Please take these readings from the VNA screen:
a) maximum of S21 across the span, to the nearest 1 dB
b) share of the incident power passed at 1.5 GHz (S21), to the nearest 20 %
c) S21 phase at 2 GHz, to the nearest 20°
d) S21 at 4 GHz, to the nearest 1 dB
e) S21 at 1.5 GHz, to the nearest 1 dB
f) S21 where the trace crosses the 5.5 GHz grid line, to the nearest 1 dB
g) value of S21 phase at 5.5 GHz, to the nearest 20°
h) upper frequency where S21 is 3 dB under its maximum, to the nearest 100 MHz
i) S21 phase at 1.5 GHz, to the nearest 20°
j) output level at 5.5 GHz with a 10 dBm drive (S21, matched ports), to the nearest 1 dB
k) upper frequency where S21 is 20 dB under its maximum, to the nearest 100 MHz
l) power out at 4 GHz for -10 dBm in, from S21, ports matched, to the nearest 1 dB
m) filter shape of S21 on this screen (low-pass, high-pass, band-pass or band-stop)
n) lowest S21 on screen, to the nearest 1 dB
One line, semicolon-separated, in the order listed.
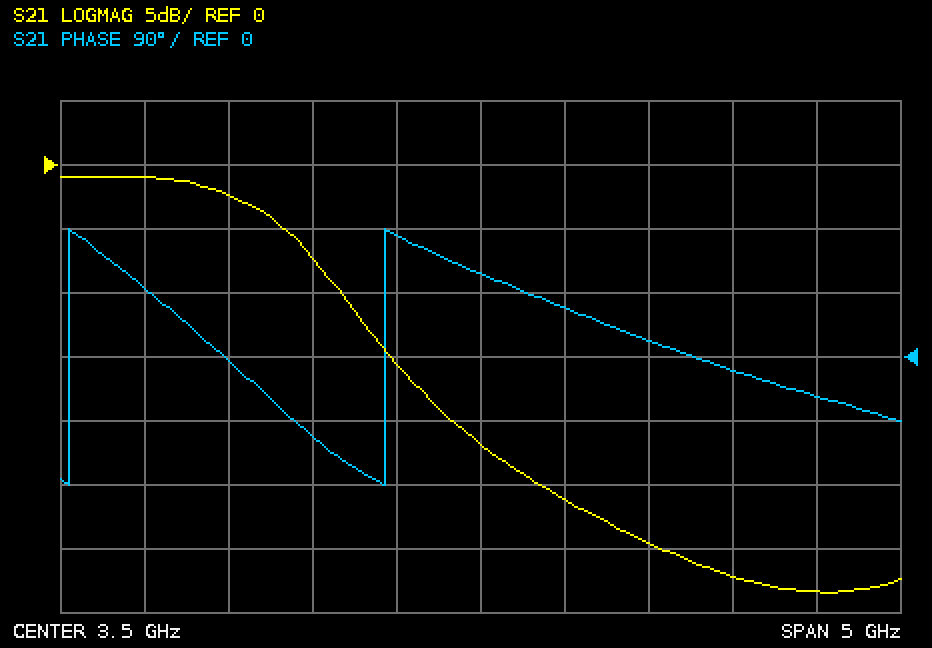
-1 dB; 80 %; 0°; -26 dB; -1 dB; -33 dB; -60°; 2.2 GHz; 100°; -23 dBm; 3.4 GHz; -36 dBm; low-pass; -33 dB
